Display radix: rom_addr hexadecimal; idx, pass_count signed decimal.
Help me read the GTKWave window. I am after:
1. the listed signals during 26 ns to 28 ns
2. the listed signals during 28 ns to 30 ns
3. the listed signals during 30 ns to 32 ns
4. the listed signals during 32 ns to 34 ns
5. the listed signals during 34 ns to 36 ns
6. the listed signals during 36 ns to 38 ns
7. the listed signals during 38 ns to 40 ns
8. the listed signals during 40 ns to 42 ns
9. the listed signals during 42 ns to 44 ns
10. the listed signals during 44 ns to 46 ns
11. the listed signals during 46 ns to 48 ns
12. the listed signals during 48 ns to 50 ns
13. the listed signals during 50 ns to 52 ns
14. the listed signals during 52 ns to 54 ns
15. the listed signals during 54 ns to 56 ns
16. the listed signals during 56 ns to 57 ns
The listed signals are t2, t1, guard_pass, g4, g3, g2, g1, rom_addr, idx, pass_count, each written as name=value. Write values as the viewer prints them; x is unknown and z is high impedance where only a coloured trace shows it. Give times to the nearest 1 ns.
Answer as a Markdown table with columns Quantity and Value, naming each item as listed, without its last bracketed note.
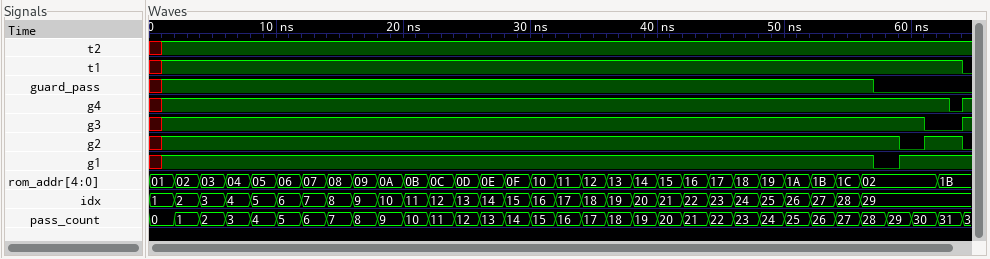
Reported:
| Quantity | Value |
|---|---|
| the listed signals during 26 ns to 28 ns | t2=1, t1=1, guard_pass=1, g4=1, g3=1, g2=1, g1=1, rom_addr=0E, idx=14, pass_count=13 |
| the listed signals during 28 ns to 30 ns | t2=1, t1=1, guard_pass=1, g4=1, g3=1, g2=1, g1=1, rom_addr=0F, idx=15, pass_count=14 |
| the listed signals during 30 ns to 32 ns | t2=1, t1=1, guard_pass=1, g4=1, g3=1, g2=1, g1=1, rom_addr=10, idx=16, pass_count=15 |
| the listed signals during 32 ns to 34 ns | t2=1, t1=1, guard_pass=1, g4=1, g3=1, g2=1, g1=1, rom_addr=11, idx=17, pass_count=16 |
| the listed signals during 34 ns to 36 ns | t2=1, t1=1, guard_pass=1, g4=1, g3=1, g2=1, g1=1, rom_addr=12, idx=18, pass_count=17 |
| the listed signals during 36 ns to 38 ns | t2=1, t1=1, guard_pass=1, g4=1, g3=1, g2=1, g1=1, rom_addr=13, idx=19, pass_count=18 |
| the listed signals during 38 ns to 40 ns | t2=1, t1=1, guard_pass=1, g4=1, g3=1, g2=1, g1=1, rom_addr=14, idx=20, pass_count=19 |
| the listed signals during 40 ns to 42 ns | t2=1, t1=1, guard_pass=1, g4=1, g3=1, g2=1, g1=1, rom_addr=15, idx=21, pass_count=20 |
| the listed signals during 42 ns to 44 ns | t2=1, t1=1, guard_pass=1, g4=1, g3=1, g2=1, g1=1, rom_addr=16, idx=22, pass_count=21 |
| the listed signals during 44 ns to 46 ns | t2=1, t1=1, guard_pass=1, g4=1, g3=1, g2=1, g1=1, rom_addr=17, idx=23, pass_count=22 |
| the listed signals during 46 ns to 48 ns | t2=1, t1=1, guard_pass=1, g4=1, g3=1, g2=1, g1=1, rom_addr=18, idx=24, pass_count=23 |
| the listed signals during 48 ns to 50 ns | t2=1, t1=1, guard_pass=1, g4=1, g3=1, g2=1, g1=1, rom_addr=19, idx=25, pass_count=24 |
| the listed signals during 50 ns to 52 ns | t2=1, t1=1, guard_pass=1, g4=1, g3=1, g2=1, g1=1, rom_addr=1A, idx=26, pass_count=25 |
| the listed signals during 52 ns to 54 ns | t2=1, t1=1, guard_pass=1, g4=1, g3=1, g2=1, g1=1, rom_addr=1B, idx=27, pass_count=26 |
| the listed signals during 54 ns to 56 ns | t2=1, t1=1, guard_pass=1, g4=1, g3=1, g2=1, g1=1, rom_addr=1C, idx=28, pass_count=27 |
| the listed signals during 56 ns to 57 ns | t2=1, t1=1, guard_pass=1, g4=1, g3=1, g2=1, g1=1, rom_addr=02, idx=29, pass_count=28 |
